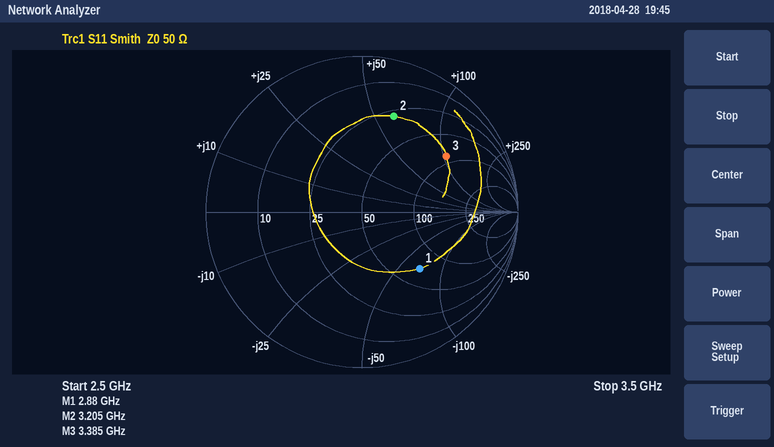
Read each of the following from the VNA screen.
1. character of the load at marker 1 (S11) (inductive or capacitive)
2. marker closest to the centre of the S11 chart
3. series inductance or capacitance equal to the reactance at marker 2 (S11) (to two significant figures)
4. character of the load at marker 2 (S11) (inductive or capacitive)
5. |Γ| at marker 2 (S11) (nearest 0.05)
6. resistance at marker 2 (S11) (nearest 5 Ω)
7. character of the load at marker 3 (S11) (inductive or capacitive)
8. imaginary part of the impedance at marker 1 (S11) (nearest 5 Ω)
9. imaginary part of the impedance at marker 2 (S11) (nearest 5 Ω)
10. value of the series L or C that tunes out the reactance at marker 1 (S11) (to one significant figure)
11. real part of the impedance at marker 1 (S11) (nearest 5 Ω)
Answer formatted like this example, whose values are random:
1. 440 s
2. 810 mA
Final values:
1. capacitive
2. marker 1
3. 3.0 nH
4. inductive
5. 0.65
6. 30 Ω
7. inductive
8. -70 Ω
9. +60 Ω
10. 4 nH
11. 70 Ω
